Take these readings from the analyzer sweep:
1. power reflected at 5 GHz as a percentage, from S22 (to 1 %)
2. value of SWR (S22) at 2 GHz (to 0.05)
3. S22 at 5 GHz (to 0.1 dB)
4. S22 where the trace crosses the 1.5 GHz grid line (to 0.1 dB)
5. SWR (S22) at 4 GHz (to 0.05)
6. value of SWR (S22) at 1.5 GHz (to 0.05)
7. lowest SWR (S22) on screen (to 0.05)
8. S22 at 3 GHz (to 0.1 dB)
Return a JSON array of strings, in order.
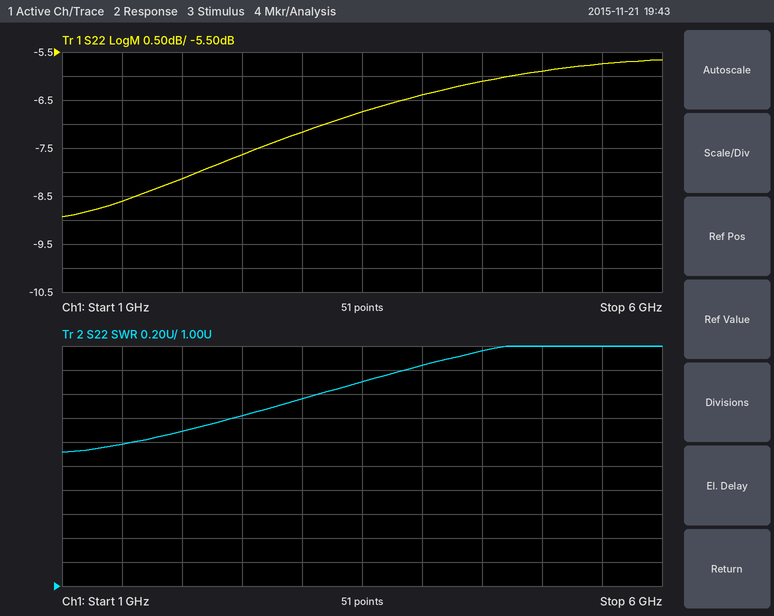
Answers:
["26 %", "2.30", "-5.9 dB", "-8.6 dB", "2.85", "2.20", "2.10", "-7.2 dB"]
